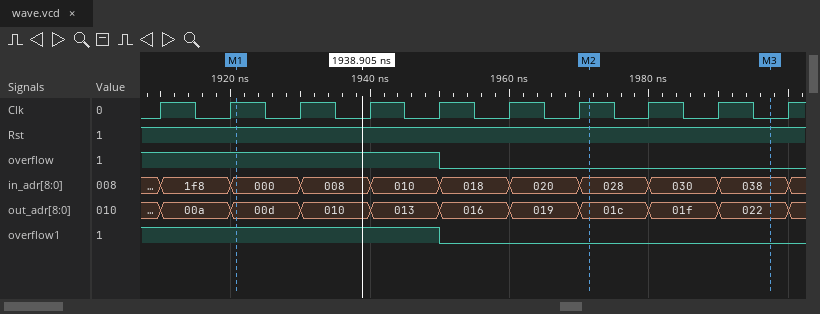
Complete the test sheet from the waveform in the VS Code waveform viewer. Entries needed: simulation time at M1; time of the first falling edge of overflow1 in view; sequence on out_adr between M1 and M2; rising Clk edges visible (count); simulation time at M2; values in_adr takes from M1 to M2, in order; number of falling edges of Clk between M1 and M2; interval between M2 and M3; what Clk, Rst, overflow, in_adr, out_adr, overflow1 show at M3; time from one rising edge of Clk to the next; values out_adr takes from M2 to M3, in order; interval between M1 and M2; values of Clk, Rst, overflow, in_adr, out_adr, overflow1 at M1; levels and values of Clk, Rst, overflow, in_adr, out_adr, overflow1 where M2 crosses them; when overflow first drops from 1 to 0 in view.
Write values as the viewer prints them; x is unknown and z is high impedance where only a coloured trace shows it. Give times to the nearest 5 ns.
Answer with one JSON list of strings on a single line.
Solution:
["1920 ns", "1950 ns", "00d, 010, 013, 016, 019, 01c", "10", "1970 ns", "000, 008, 010, 018, 020, 028", "5", "25 ns", "Clk=0, Rst=1, overflow=0, in_adr=038, out_adr=022, overflow1=0", "10 ns", "01c, 01f, 022", "50 ns", "Clk=1, Rst=1, overflow=1, in_adr=000, out_adr=00d, overflow1=1", "Clk=1, Rst=1, overflow=0, in_adr=028, out_adr=01c, overflow1=0", "1950 ns"]
